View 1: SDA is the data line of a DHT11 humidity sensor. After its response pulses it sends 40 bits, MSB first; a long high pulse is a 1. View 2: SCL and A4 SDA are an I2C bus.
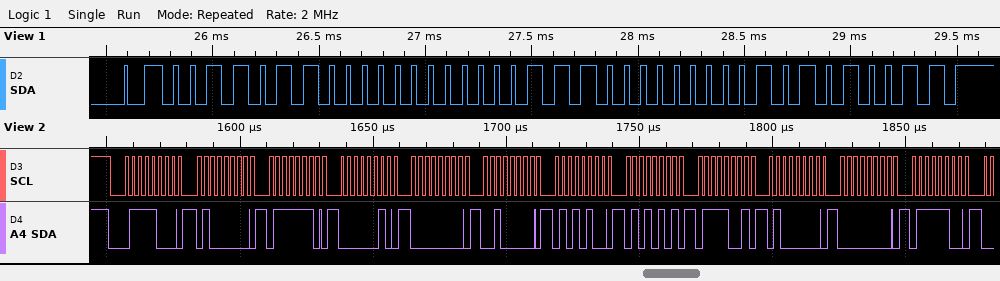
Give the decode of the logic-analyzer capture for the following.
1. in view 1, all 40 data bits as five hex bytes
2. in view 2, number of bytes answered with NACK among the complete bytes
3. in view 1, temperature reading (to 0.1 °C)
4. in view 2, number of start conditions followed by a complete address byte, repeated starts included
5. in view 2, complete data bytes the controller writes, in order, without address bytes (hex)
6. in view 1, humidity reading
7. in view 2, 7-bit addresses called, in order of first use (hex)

36 00 1C 01 53
0
28.1 °C
1
40 7E 02 00 20 54 55 79 40 00 7C
54 %
0x3C
